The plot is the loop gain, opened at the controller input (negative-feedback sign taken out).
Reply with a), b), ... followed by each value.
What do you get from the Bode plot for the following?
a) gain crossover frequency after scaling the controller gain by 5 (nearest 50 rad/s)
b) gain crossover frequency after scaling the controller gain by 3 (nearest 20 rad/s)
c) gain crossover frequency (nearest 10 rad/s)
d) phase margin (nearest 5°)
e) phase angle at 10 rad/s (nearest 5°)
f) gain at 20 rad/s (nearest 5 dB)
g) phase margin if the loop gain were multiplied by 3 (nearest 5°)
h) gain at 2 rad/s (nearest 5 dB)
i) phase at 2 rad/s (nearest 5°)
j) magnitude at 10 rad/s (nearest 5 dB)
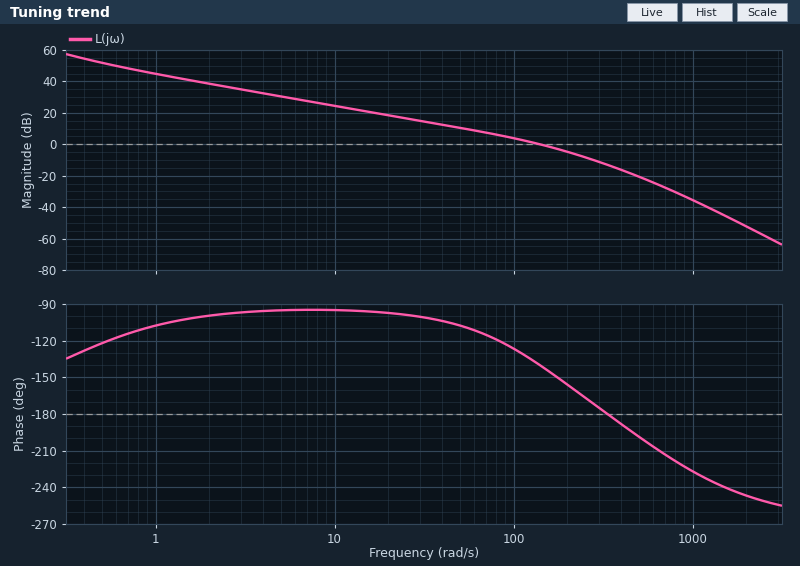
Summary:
a) 350 rad/s
b) 280 rad/s
c) 140 rad/s
d) 40°
e) -95°
f) 20 dB
g) 10°
h) 40 dB
i) -100°
j) 25 dB
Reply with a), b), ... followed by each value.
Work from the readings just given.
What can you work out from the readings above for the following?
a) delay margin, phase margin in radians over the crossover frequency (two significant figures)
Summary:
a) 0.0050 s
